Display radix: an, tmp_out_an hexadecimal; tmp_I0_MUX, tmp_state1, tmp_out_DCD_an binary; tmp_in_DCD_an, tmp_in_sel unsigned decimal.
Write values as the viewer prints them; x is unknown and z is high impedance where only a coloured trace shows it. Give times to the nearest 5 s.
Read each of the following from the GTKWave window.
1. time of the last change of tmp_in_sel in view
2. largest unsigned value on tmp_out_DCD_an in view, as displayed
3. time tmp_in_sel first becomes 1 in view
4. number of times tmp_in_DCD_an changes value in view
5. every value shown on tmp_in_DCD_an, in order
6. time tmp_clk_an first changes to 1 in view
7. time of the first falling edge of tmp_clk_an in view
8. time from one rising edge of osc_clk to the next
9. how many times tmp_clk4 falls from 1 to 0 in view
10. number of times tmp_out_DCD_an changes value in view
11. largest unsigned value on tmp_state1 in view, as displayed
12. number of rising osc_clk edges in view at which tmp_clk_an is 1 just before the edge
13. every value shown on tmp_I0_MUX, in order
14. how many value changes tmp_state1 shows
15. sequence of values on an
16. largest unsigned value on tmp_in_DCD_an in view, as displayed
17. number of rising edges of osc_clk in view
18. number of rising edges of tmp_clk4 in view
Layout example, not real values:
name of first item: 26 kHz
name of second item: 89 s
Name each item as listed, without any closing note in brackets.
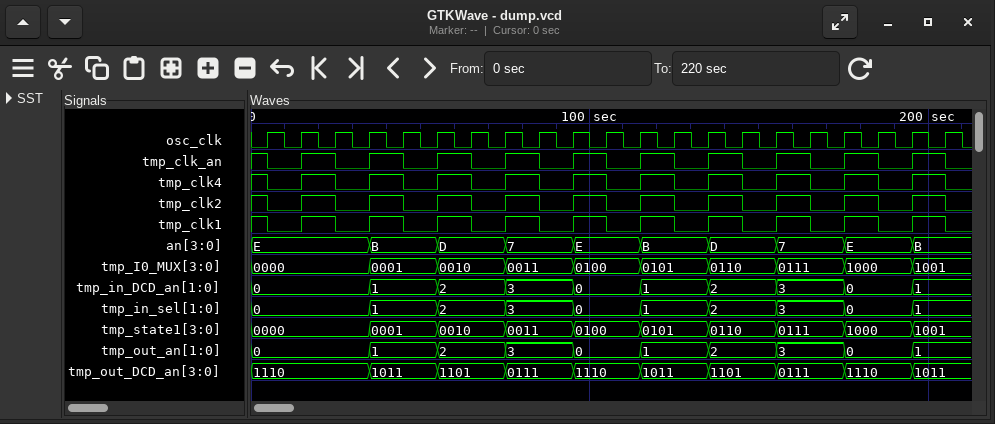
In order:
time of the last change of tmp_in_sel in view: 195 s
largest unsigned value on tmp_out_DCD_an in view, as displayed: 1110
time tmp_in_sel first becomes 1 in view: 35 s
number of times tmp_in_DCD_an changes value in view: 9
every value shown on tmp_in_DCD_an, in order: 0, 1, 2, 3, 0, 1, 2, 3, 0, 1
time tmp_clk_an first changes to 1 in view: 15 s
time of the first falling edge of tmp_clk_an in view: 5 s
time from one rising edge of osc_clk to the next: 10 s
how many times tmp_clk4 falls from 1 to 0 in view: 11
number of times tmp_out_DCD_an changes value in view: 9
largest unsigned value on tmp_state1 in view, as displayed: 1001
number of rising osc_clk edges in view at which tmp_clk_an is 1 just before the edge: 11
every value shown on tmp_I0_MUX, in order: 0000, 0001, 0010, 0011, 0100, 0101, 0110, 0111, 1000, 1001
how many value changes tmp_state1 shows: 9
sequence of values on an: E, B, D, 7, E, B, D, 7, E, B
largest unsigned value on tmp_in_DCD_an in view, as displayed: 3
number of rising edges of osc_clk in view: 21
number of rising edges of tmp_clk4 in view: 10
